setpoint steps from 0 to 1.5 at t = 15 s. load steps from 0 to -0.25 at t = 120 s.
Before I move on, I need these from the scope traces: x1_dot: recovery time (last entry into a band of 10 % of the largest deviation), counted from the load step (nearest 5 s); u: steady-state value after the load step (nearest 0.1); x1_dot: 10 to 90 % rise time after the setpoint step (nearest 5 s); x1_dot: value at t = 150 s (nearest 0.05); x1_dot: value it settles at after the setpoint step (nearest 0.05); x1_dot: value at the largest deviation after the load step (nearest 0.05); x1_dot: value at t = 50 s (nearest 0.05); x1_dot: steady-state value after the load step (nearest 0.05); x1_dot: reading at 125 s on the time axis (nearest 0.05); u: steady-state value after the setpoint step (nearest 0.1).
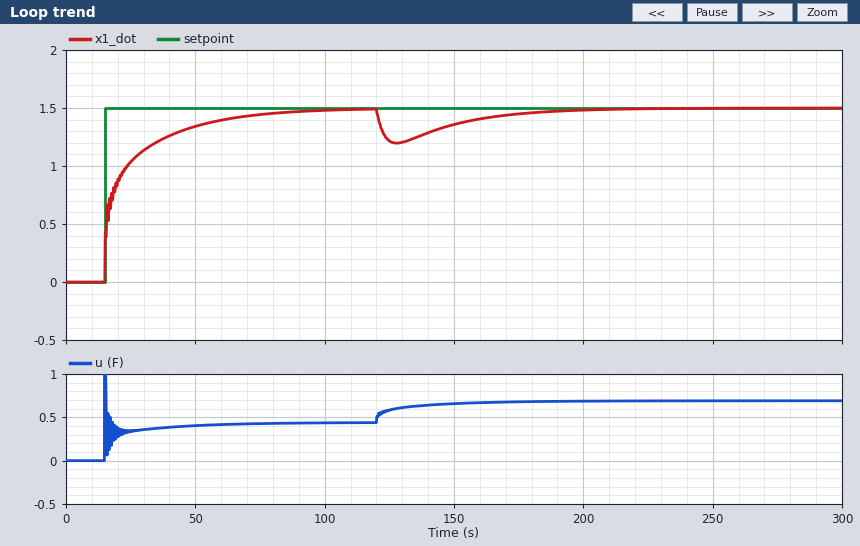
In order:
70 s
0.7
35 s
1.35
1.50
1.20
1.35
1.50
1.20
0.4
